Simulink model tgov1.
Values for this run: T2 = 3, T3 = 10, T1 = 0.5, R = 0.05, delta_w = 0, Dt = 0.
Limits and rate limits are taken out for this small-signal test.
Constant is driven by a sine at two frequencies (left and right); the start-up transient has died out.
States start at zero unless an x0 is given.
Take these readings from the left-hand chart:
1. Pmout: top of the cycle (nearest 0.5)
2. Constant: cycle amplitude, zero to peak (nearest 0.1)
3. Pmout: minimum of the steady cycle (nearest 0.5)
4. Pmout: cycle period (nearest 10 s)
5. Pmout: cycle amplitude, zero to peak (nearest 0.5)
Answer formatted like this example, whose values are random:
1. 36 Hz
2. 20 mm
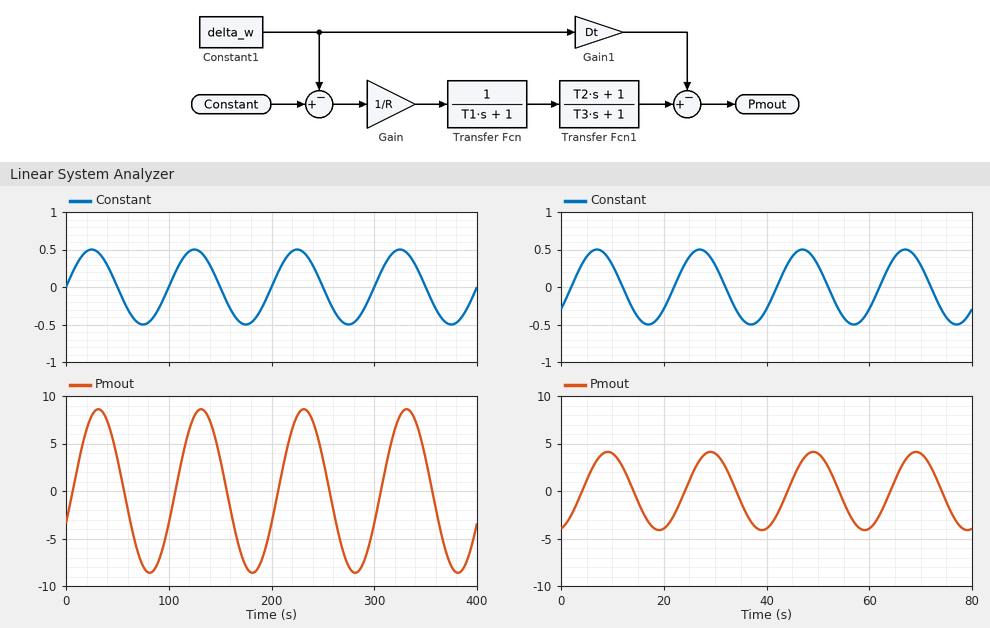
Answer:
1. 8.5
2. 0.5
3. -8.5
4. 100 s
5. 8.5
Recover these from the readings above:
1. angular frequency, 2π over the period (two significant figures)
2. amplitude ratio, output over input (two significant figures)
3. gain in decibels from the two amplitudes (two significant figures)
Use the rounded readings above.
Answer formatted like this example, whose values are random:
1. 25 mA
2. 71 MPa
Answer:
1. 0.063 rad/s
2. 17
3. 25 dB
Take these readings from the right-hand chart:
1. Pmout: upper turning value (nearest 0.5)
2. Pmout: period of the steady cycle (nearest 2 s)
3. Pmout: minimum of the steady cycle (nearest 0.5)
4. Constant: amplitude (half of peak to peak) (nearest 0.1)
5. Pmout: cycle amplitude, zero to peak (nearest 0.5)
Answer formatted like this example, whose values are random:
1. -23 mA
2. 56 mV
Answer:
1. 4.0
2. 20 s
3. -4.0
4. 0.5
5. 4.0
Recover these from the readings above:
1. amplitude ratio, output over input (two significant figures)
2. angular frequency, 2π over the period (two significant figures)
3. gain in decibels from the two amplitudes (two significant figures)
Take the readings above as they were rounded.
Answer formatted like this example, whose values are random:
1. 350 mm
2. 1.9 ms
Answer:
1. 8.0
2. 0.31 rad/s
3. 18 dB
